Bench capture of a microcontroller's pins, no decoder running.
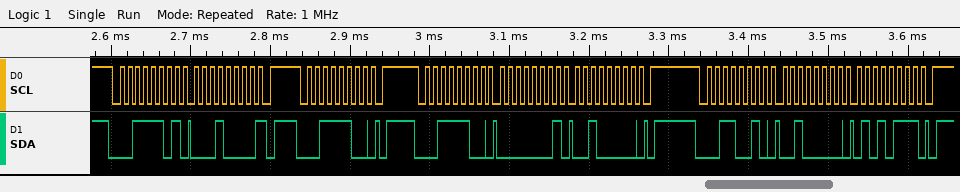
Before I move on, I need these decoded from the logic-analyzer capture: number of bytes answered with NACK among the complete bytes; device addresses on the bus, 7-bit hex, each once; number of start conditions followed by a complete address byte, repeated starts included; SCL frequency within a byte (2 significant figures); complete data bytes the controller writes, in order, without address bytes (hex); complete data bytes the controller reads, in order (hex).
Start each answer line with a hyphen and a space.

- 1
- 0x1E 0x19
- 4
- 100 kHz
- 01 20 20 57
- 10
